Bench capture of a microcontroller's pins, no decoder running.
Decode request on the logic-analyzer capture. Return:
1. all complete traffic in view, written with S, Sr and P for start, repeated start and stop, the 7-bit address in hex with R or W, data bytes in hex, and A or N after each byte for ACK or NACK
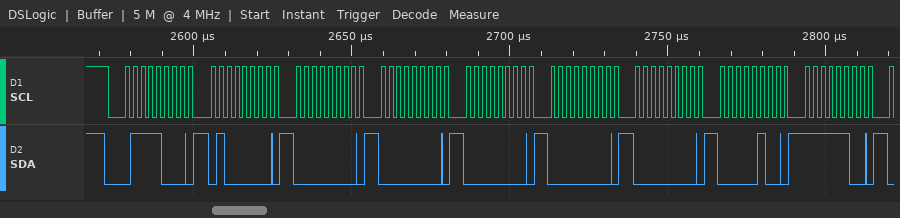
S 3CW A 40 A 00 A 00 A 00 A 00 A 00 A 04 A FC A
